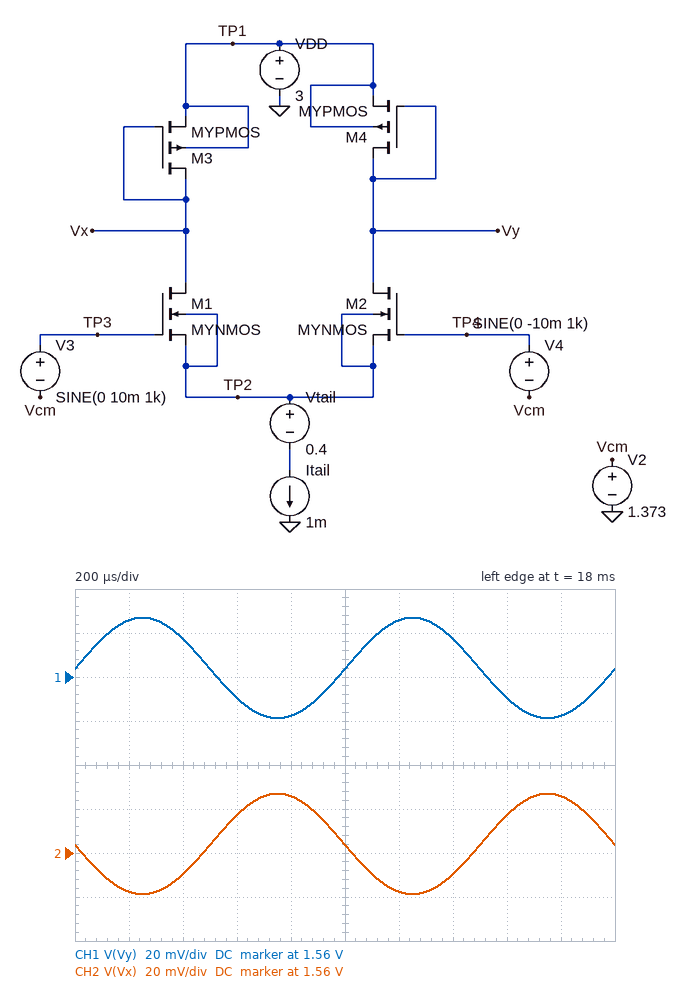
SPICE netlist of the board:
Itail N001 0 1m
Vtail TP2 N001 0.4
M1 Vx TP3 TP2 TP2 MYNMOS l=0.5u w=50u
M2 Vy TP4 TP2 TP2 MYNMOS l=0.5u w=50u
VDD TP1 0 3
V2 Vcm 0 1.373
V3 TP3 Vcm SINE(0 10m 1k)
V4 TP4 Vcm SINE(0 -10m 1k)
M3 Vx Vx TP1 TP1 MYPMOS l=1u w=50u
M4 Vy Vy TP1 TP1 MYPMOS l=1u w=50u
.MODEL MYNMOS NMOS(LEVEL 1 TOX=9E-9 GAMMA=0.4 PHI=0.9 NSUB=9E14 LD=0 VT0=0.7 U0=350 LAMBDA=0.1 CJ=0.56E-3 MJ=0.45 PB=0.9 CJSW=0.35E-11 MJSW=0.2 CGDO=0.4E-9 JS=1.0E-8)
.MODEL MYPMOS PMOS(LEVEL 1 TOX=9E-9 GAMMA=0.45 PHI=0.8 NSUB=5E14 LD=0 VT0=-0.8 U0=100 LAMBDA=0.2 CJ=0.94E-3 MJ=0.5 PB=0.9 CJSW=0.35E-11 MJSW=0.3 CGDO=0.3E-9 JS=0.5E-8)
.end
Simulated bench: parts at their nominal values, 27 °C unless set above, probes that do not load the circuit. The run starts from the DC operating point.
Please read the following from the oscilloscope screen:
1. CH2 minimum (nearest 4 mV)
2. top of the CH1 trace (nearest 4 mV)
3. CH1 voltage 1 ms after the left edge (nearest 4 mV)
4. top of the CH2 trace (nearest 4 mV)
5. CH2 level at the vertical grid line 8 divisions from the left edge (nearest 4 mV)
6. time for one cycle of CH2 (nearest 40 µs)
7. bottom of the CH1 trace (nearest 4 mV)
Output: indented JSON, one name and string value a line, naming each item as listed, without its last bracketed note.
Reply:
{
  "CH2 minimum": "1.540 V",
  "top of the CH1 trace": "1.588 V",
  "CH1 voltage 1 ms after the left edge": "1.564 V",
  "top of the CH2 trace": "1.588 V",
  "CH2 level at the vertical grid line 8 divisions from the left edge": "1.576 V",
  "time for one cycle of CH2": "1.00 ms",
  "bottom of the CH1 trace": "1.540 V"
}
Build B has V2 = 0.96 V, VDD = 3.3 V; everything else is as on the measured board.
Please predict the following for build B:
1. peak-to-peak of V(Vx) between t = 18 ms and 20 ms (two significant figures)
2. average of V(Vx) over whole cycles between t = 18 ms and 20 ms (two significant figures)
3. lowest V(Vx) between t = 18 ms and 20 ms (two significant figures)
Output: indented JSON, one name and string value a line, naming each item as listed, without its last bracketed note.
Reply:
{
  "peak-to-peak of V(Vx) between t = 18 ms and 20 ms": "47 mV",
  "average of V(Vx) over whole cycles between t = 18 ms and 20 ms": "1.9 V",
  "lowest V(Vx) between t = 18 ms and 20 ms": "1.8 V"
}
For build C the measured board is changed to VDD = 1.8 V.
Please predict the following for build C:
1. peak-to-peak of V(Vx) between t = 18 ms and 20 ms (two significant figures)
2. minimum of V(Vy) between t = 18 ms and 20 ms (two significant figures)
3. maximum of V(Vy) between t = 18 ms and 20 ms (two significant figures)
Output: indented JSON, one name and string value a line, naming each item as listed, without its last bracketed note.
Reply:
{
  "peak-to-peak of V(Vx) between t = 18 ms and 20 ms": "4.7 mV",
  "minimum of V(Vy) between t = 18 ms and 20 ms": "360 mV",
  "maximum of V(Vy) between t = 18 ms and 20 ms": "370 mV"
}
